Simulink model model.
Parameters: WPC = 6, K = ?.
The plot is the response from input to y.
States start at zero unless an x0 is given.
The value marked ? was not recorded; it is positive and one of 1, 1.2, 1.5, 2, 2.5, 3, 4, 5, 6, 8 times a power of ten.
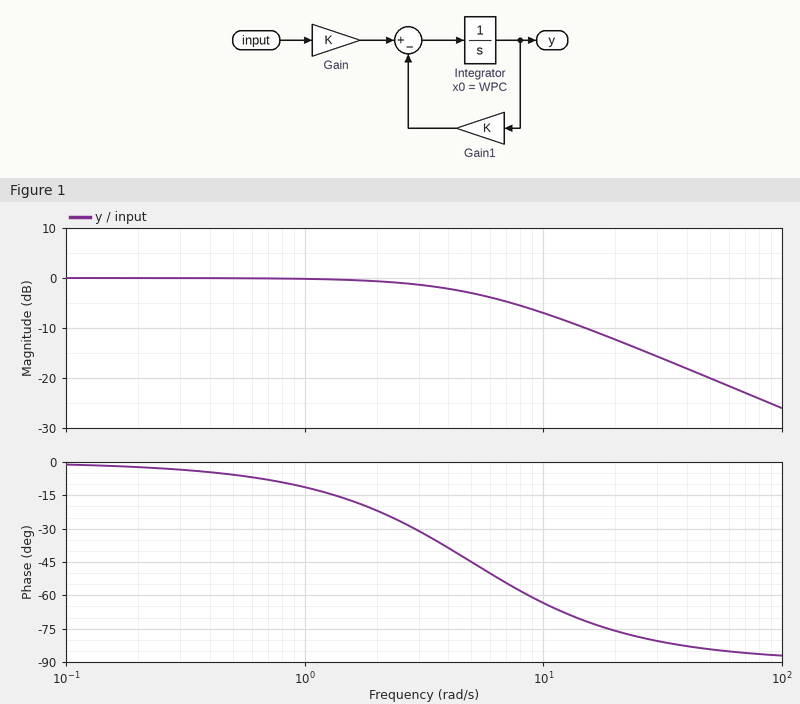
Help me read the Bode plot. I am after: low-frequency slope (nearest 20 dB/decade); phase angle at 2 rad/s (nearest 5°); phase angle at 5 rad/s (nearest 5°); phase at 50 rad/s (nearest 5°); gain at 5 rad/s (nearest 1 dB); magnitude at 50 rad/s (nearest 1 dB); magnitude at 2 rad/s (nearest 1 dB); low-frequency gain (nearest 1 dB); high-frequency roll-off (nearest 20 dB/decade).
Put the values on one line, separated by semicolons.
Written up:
0 dB/decade; -20°; -45°; -85°; -3 dB; -20 dB; -1 dB; 0 dB; -20 dB/decade
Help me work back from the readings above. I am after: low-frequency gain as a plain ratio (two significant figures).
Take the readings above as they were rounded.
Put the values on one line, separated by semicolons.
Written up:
1.0
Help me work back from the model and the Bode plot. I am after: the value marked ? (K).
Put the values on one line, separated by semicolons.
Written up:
5
